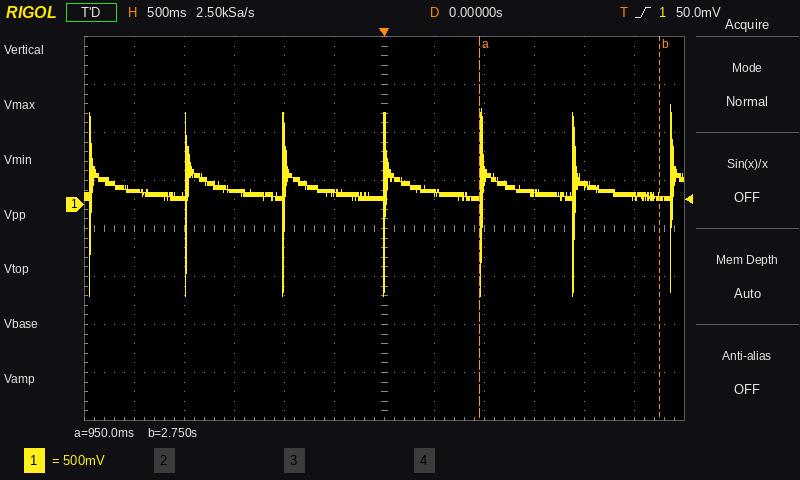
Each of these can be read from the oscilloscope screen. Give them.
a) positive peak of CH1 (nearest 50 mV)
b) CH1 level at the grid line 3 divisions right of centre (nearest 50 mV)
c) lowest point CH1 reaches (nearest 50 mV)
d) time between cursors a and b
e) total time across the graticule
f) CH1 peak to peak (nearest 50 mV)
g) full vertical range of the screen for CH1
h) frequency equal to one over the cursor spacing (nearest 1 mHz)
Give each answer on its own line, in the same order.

1.05 V
100 mV
-950 mV
1.80 s
6 s
2.00 V
4 V
556 mHz
